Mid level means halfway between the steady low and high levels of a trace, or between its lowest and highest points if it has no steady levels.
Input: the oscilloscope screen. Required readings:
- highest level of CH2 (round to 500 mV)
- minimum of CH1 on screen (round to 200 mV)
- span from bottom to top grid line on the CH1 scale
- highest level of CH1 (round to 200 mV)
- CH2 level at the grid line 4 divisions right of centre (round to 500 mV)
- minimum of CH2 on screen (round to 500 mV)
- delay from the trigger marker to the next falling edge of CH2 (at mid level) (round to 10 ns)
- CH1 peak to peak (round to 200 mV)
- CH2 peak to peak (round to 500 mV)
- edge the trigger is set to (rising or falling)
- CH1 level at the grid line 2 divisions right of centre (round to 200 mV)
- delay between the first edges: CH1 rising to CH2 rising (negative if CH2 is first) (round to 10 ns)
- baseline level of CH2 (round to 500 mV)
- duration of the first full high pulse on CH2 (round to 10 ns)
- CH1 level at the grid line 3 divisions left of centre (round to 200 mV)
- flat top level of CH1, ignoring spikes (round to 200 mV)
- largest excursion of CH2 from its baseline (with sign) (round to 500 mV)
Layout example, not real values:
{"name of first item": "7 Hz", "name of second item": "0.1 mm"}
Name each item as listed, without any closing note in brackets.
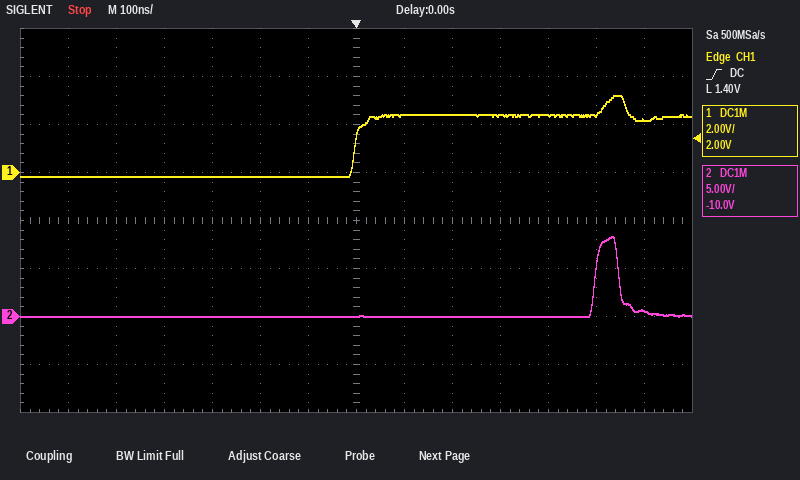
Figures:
{"highest level of CH2": "8.5 V", "minimum of CH1 on screen": "-200 mV", "span from bottom to top grid line on the CH1 scale": "16 V", "highest level of CH1": "3.2 V", "CH2 level at the grid line 4 divisions right of centre": "0.0 V", "minimum of CH2 on screen": "0.0 V", "delay from the trigger marker to the next falling edge of CH2 (at mid level)": "550 ns", "CH1 peak to peak": "3.4 V", "CH2 peak to peak": "8.5 V", "edge the trigger is set to": "rising", "CH1 level at the grid line 2 divisions right of centre": "2.4 V", "delay between the first edges: CH1 rising to CH2 rising (negative if CH2 is first)": "+500 ns", "baseline level of CH2": "0.0 V", "duration of the first full high pulse on CH2": "50 ns", "CH1 level at the grid line 3 divisions left of centre": "-200 mV", "flat top level of CH1, ignoring spikes": "2.4 V", "largest excursion of CH2 from its baseline (with sign)": "+8.5 V"}
